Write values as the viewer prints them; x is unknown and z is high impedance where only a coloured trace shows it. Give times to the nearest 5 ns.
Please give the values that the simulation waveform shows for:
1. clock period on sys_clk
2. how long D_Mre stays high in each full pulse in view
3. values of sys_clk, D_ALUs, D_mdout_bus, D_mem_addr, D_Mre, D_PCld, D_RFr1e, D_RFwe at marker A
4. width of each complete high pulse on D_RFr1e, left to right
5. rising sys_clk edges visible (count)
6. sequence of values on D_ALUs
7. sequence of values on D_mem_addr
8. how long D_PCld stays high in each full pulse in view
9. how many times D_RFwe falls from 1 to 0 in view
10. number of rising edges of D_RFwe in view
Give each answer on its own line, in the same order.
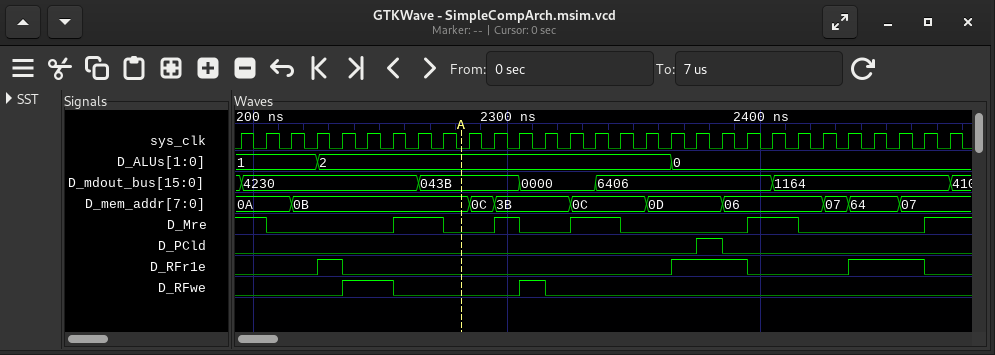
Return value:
10 ns
20 ns, 10 ns, 20 ns, 20 ns
sys_clk=0, D_ALUs=2, D_mdout_bus=043B, D_mem_addr=0B, D_Mre=0, D_PCld=0, D_RFr1e=0, D_RFwe=0
10 ns, 30 ns, 30 ns
29
1, 2, 0
0A, 0B, 0C, 3B, 0C, 0D, 06, 07, 64, 07
10 ns
2
2
